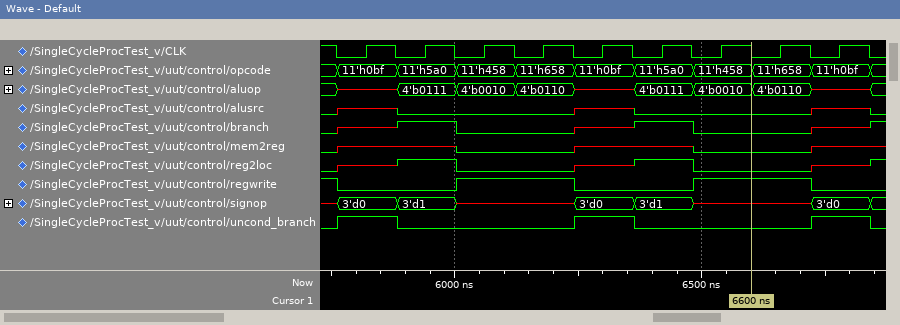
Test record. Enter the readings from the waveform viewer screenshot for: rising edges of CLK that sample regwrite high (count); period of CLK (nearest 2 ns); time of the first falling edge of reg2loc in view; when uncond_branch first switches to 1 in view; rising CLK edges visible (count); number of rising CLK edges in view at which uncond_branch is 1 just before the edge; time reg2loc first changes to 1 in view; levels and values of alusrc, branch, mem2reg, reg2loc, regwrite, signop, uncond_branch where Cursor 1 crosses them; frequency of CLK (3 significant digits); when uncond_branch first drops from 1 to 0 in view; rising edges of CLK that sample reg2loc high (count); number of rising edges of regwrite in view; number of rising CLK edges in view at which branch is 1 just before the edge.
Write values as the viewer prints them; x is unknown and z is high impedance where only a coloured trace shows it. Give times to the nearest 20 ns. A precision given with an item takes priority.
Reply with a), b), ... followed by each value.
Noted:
a) 4
b) 120 ns
c) 6000 ns
d) 5760 ns
e) 9
f) 3
g) 5880 ns
h) alusrc=0, branch=0, mem2reg=0, reg2loc=0, regwrite=1, signop=x, uncond_branch=0
i) 8.33 MHz
j) 5880 ns
k) 2
l) 2
m) 2
